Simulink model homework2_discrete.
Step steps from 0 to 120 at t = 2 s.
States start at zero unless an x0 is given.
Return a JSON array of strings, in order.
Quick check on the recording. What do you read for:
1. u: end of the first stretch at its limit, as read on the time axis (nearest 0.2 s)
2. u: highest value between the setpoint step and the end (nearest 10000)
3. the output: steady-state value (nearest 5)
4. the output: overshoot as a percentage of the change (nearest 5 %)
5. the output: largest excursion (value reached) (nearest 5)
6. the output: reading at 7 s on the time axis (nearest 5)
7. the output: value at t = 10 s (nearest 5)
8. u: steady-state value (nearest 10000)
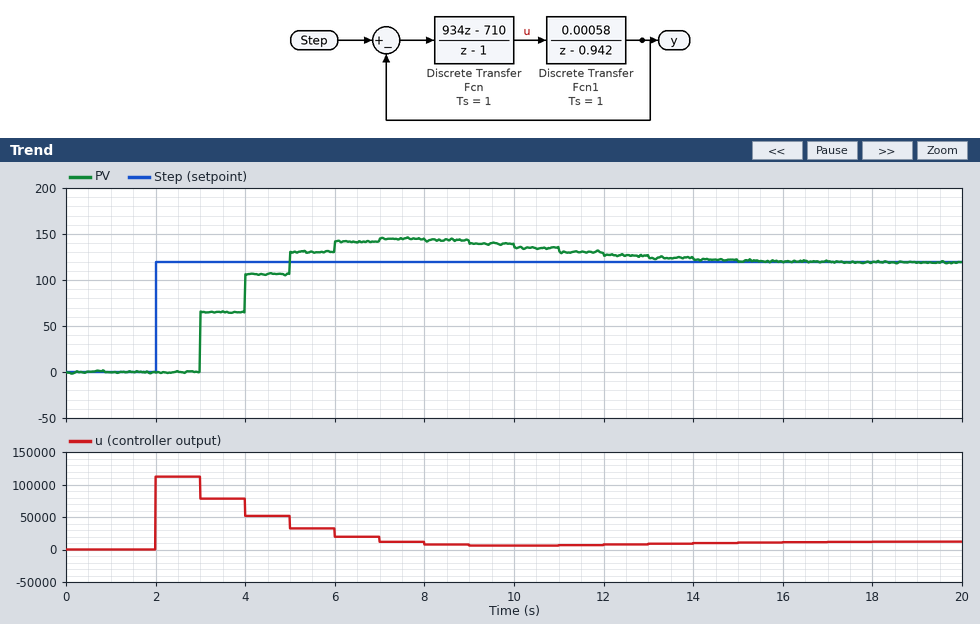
["3.0 s", "110000", "120", "20 %", "145", "145", "135", "10000"]
